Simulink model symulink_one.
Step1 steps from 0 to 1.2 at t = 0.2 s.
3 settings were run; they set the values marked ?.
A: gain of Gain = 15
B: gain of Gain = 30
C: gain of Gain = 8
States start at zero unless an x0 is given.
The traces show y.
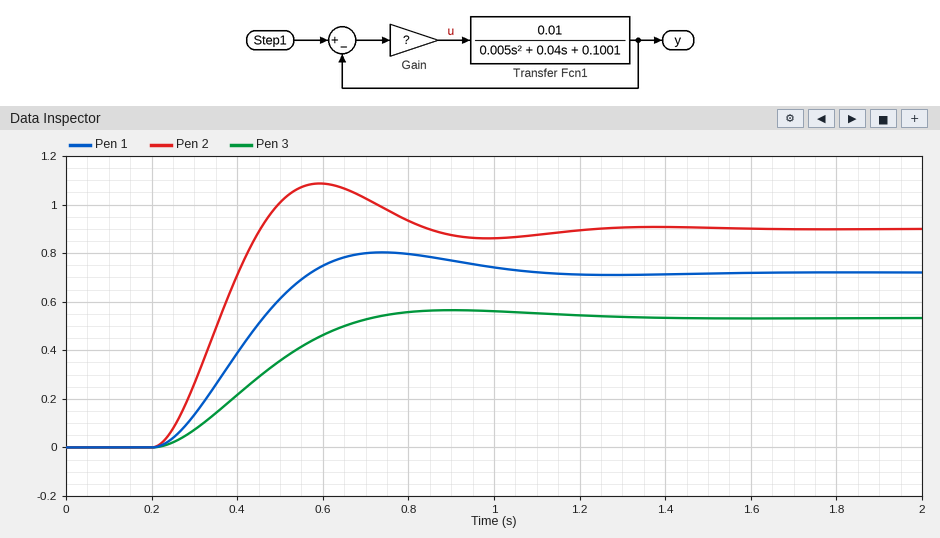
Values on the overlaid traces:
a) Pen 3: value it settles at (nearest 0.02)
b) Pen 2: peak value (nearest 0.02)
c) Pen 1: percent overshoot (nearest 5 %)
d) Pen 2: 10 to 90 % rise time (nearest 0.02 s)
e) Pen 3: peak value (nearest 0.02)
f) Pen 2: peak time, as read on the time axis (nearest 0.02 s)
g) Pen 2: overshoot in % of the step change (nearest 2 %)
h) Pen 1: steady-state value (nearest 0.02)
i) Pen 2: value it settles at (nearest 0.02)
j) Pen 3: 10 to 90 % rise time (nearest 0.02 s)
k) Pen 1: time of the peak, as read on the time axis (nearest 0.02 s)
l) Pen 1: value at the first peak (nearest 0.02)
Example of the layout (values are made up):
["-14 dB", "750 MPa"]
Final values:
["0.54", "1.08", "10 %", "0.18 s", "0.56", "0.60 s", "20 %", "0.72", "0.90", "0.34 s", "0.74 s", "0.80"]
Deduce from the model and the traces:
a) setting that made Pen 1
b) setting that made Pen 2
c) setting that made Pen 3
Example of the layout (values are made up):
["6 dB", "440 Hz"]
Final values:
["A", "B", "C"]
